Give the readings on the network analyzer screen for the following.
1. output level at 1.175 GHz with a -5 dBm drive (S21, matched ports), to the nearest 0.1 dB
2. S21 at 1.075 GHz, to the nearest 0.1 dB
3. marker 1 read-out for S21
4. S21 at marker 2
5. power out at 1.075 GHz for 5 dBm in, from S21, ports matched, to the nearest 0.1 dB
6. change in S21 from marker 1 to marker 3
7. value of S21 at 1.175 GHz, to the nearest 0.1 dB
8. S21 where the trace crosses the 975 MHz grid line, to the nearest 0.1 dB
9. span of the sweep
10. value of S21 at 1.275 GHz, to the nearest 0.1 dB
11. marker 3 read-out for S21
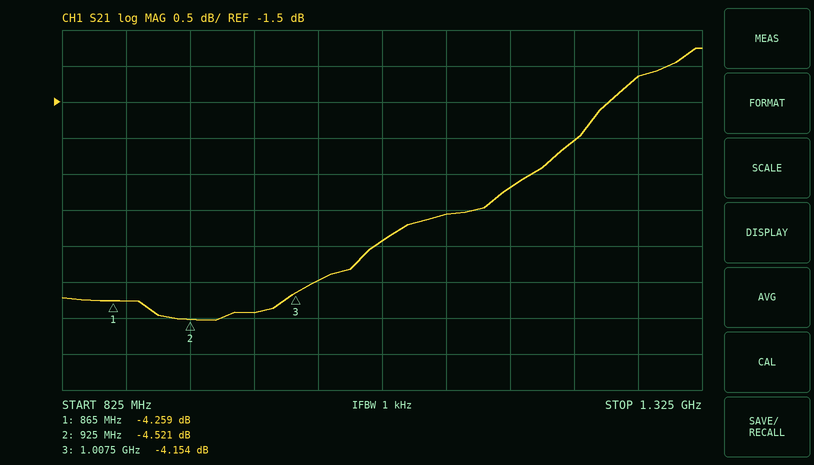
-7.7 dBm
-3.4 dB
-4.259 dB
-4.521 dB
1.6 dBm
0.105 dB
-2.7 dB
-4.4 dB
500 MHz
-1.1 dB
-4.154 dB
